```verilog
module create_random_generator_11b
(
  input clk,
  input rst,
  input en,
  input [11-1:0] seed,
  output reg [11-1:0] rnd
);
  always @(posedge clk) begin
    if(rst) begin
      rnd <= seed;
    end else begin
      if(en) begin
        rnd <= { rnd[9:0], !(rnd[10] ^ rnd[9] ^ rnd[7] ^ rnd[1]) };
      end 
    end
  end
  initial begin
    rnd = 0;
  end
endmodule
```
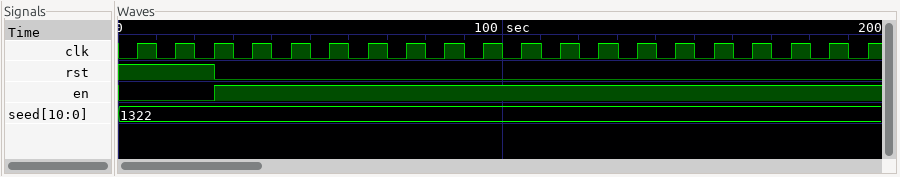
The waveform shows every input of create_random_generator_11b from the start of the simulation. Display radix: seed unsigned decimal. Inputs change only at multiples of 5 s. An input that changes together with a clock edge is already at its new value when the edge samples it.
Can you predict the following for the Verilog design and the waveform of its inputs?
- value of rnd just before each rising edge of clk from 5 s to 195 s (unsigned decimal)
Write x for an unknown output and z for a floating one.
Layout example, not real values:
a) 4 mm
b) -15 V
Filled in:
a) 0, 1322, 1322, 597, 1194, 340, 681, 1363, 679, 1358, 669, 1339, 631, 1263, 478, 957, 1915, 1782, 1517, 987
